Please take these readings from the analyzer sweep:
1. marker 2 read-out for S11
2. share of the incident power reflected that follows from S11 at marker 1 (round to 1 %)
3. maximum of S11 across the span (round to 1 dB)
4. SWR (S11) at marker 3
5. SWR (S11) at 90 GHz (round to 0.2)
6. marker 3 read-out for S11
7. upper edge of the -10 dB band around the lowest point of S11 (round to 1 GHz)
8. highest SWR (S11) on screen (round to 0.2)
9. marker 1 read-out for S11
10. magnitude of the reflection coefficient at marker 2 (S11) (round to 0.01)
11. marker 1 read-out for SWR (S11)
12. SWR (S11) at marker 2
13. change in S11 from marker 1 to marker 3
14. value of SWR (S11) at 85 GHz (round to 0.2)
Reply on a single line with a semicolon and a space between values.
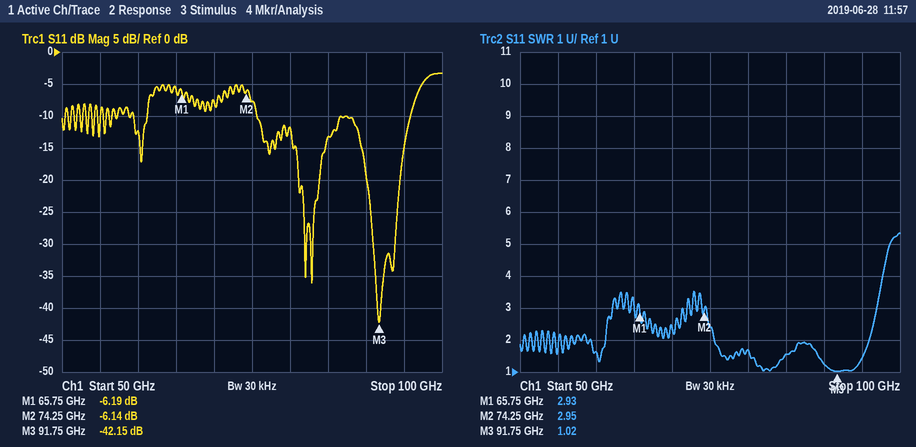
-6.14 dB; 24 %; -3 dB; 1.02; 1.2; -42.15 dB; 96 GHz; 5.4; -6.19 dB; 0.49; 2.93; 2.95; -35.96 dB; 1.6
